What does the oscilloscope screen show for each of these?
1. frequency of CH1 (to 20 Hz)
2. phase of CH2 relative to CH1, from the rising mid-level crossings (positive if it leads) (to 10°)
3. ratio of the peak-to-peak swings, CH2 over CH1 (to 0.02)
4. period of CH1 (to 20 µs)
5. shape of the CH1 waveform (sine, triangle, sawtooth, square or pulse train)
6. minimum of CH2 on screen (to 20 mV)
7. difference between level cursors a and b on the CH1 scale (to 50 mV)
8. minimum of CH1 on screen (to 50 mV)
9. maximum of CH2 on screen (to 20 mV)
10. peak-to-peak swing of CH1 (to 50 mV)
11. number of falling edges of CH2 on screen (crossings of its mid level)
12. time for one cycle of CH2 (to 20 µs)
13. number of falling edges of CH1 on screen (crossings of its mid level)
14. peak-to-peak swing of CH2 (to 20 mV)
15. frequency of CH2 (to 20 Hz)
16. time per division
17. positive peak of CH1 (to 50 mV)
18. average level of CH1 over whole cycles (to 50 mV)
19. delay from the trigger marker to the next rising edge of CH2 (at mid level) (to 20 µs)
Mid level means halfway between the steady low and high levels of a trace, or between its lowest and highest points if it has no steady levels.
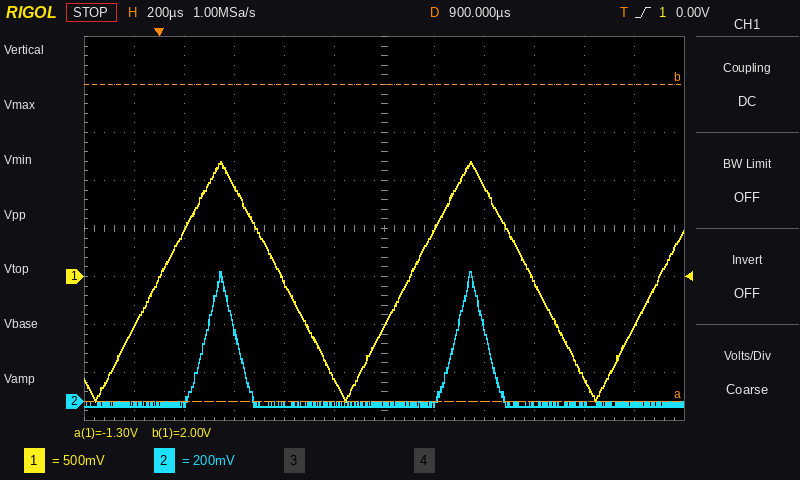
1.00 kHz
-70°
0.22
1.00 ms
triangle
-20 mV
3.30 V
-1.30 V
540 mV
2.50 V
2
1.00 ms
2
560 mV
1.00 kHz
200 µs
1.20 V
-50 mV
180 µs
